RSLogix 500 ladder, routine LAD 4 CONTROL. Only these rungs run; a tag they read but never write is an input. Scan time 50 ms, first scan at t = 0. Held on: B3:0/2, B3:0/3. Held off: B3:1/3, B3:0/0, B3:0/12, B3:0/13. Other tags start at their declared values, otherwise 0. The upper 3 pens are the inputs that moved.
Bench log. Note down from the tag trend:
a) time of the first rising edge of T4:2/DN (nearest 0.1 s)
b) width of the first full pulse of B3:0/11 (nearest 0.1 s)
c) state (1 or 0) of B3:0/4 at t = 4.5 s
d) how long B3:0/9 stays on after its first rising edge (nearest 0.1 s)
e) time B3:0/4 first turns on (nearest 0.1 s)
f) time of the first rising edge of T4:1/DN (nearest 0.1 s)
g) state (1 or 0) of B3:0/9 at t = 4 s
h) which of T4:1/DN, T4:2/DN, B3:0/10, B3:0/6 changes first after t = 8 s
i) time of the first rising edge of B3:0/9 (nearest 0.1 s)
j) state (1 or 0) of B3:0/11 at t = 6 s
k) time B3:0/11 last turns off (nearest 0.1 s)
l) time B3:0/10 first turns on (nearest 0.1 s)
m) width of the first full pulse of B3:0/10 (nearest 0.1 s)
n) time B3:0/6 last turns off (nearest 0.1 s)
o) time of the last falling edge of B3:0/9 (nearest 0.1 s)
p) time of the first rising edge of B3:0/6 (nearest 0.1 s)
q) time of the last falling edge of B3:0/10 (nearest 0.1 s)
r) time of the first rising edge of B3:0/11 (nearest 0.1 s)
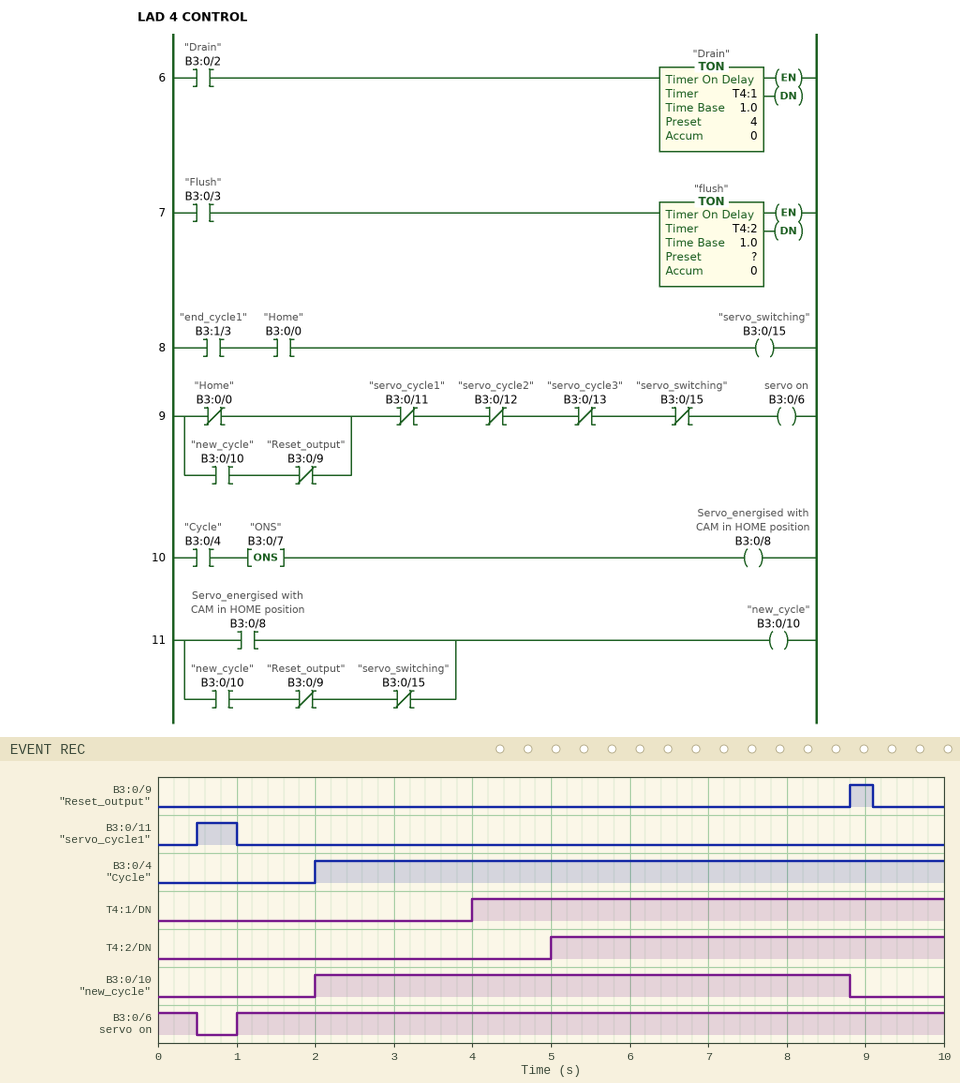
5.0 s
0.5 s
1
0.3 s
2.0 s
4.0 s
0
B3:0/10
8.8 s
0
1.0 s
2.0 s
6.8 s
0.5 s
9.1 s
1.0 s
8.8 s
0.5 s
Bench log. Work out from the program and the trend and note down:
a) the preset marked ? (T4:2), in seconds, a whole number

5 s
